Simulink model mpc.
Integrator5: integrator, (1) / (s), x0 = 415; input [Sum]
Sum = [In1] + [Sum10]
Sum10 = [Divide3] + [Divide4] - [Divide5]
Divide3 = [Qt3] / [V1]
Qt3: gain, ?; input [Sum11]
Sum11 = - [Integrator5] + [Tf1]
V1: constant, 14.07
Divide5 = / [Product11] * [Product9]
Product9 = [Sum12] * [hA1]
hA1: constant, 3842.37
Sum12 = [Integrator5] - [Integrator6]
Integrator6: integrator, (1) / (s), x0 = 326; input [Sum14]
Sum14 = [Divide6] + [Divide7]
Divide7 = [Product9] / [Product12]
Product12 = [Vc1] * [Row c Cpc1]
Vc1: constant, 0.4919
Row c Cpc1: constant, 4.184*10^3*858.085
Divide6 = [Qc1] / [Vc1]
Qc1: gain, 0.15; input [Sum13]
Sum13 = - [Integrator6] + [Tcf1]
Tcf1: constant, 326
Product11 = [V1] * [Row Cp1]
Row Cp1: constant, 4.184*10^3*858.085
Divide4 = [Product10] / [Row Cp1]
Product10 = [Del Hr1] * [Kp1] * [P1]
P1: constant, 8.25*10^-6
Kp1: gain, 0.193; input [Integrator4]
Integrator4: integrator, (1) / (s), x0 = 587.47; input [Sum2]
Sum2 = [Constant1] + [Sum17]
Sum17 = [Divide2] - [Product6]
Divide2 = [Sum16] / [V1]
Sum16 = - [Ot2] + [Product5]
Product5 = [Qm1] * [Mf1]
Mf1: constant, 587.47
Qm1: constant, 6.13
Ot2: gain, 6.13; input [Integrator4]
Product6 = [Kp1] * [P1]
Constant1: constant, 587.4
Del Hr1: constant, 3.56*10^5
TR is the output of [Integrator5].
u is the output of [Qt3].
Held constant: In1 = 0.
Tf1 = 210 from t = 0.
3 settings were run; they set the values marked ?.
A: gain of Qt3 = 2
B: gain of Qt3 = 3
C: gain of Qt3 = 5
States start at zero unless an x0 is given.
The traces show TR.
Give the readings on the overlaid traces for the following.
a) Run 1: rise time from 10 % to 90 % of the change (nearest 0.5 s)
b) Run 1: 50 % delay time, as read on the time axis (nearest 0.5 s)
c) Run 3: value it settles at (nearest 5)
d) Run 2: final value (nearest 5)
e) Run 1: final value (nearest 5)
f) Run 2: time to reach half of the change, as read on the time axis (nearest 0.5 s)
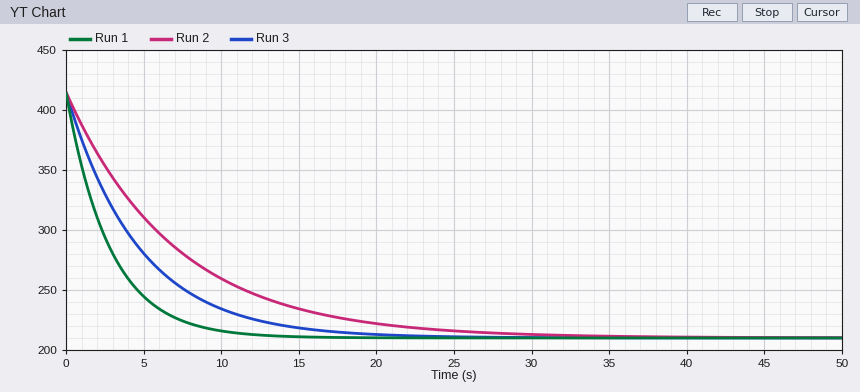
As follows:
6.0 s
2.0 s
210
210
210
5.0 s
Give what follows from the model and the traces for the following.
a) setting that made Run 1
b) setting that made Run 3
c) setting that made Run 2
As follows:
C
B
A
